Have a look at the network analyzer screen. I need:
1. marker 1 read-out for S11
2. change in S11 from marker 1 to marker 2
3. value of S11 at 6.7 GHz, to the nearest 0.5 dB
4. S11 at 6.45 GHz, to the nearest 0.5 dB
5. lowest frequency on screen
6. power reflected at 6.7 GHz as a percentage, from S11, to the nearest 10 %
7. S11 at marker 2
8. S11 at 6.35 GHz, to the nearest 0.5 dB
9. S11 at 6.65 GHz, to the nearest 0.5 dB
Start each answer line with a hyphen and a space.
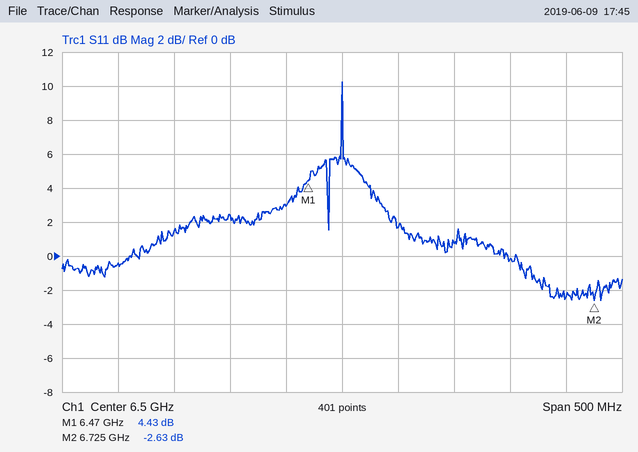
- 4.43 dB
- -7.06 dB
- -2.5 dB
- 3.0 dB
- 6.25 GHz
- 60 %
- -2.63 dB
- 1.5 dB
- 0.0 dB
